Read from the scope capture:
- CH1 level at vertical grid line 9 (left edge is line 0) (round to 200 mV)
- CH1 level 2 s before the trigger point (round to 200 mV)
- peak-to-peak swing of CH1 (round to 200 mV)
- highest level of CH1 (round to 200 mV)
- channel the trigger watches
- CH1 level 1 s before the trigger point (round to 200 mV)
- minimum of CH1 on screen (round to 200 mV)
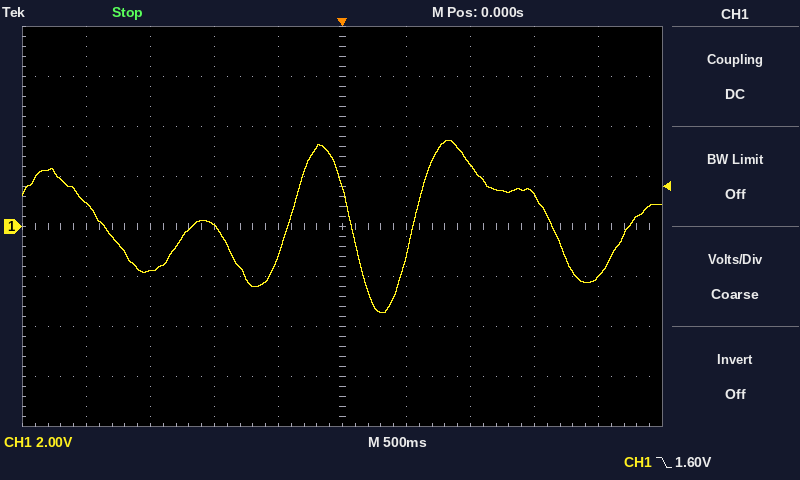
-2.0 V
1.0 V
6.8 V
3.4 V
CH1
0.0 V
-3.4 V
